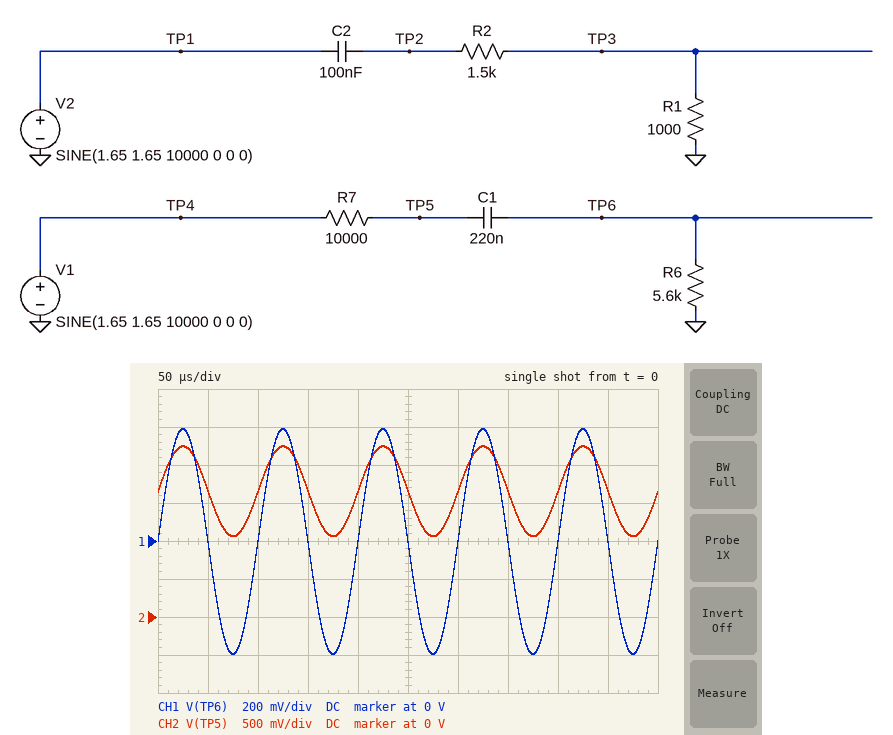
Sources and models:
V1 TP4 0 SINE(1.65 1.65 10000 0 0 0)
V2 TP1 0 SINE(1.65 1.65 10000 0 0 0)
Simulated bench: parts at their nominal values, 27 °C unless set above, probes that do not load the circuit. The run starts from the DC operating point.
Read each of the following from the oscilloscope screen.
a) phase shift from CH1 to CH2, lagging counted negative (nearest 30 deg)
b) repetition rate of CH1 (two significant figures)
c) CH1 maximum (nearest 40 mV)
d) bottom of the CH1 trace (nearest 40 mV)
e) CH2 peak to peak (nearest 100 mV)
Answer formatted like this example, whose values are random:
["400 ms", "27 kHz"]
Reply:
["0 deg", "10 kHz", "600 mV", "-600 mV", "1.2 V"]
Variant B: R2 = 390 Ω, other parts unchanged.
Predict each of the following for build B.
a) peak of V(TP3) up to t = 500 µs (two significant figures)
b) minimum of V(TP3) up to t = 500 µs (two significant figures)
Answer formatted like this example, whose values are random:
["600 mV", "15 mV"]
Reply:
["1.2 V", "-1.3 V"]
